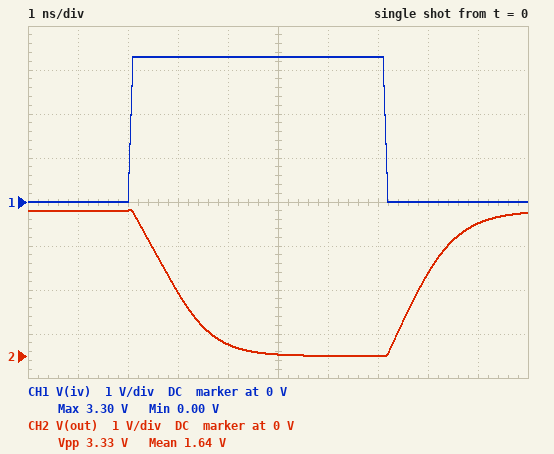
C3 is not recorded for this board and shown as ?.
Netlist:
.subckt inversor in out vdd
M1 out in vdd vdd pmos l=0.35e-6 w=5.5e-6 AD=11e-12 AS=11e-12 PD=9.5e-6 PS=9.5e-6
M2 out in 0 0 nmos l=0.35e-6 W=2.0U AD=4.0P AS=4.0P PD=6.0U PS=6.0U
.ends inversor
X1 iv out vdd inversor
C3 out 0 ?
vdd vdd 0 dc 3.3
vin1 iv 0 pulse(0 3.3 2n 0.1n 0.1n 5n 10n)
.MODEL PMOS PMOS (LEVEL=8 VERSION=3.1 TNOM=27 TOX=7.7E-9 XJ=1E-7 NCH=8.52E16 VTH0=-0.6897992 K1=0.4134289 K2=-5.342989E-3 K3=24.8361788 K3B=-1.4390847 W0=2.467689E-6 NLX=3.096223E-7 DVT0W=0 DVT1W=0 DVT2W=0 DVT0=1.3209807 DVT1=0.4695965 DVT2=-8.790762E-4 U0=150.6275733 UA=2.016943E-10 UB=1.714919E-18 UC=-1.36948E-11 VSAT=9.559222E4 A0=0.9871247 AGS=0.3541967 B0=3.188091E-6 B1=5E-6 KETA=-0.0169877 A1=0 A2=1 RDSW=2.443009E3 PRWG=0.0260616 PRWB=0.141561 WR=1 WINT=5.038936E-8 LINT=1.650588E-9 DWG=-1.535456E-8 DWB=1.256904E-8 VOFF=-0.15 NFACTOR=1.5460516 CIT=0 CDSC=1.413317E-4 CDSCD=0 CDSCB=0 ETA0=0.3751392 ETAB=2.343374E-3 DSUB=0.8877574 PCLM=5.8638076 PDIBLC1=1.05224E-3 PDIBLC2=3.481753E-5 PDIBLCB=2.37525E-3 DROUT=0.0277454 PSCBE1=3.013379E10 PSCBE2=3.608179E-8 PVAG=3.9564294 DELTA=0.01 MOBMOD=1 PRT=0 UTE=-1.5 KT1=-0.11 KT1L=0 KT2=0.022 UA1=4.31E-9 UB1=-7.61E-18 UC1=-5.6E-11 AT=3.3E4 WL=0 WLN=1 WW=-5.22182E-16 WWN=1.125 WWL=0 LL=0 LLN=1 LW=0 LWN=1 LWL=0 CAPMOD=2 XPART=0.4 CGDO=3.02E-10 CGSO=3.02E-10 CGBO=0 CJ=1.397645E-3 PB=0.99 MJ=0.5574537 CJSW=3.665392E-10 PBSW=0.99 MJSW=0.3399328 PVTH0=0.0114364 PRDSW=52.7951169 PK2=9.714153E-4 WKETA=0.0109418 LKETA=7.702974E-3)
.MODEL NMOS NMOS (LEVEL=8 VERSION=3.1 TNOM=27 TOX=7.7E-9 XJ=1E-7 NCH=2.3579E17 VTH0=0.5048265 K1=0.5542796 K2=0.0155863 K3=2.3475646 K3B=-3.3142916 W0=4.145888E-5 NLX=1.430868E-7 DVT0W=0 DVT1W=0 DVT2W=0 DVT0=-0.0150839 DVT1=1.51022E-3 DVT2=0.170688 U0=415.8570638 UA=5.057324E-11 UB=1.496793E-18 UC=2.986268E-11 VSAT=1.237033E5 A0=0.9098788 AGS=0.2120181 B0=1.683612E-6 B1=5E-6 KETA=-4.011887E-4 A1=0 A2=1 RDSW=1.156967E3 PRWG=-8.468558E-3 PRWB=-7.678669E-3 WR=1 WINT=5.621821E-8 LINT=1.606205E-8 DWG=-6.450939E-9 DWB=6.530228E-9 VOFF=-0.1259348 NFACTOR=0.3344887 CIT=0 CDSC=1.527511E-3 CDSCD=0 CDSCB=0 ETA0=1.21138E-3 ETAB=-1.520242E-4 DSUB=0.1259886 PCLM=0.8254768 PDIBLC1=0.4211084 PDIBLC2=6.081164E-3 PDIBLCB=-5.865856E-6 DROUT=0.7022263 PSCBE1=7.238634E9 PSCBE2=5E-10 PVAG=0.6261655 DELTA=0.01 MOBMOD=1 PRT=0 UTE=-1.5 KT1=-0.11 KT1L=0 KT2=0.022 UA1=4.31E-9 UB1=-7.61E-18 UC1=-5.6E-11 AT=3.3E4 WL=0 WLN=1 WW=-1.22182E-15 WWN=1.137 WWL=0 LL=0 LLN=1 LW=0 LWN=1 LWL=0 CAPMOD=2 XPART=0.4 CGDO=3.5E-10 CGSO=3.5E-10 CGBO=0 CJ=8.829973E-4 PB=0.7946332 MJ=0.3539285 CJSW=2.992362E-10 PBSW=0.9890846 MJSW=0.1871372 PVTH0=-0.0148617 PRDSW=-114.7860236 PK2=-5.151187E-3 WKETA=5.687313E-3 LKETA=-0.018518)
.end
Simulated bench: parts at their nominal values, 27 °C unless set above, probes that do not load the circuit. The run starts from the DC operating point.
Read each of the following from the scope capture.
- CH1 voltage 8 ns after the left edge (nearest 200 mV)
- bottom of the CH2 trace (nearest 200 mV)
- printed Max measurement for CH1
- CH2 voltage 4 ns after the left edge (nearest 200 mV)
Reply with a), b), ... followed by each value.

a) 0 V
b) 0 V
c) 3.30 V
d) 200 mV
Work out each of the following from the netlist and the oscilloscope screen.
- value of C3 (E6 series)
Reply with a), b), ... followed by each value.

a) 470 fF
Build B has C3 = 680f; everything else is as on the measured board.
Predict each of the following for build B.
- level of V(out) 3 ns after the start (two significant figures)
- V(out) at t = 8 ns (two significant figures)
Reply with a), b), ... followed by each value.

a) 2.0 V
b) 1.4 V
